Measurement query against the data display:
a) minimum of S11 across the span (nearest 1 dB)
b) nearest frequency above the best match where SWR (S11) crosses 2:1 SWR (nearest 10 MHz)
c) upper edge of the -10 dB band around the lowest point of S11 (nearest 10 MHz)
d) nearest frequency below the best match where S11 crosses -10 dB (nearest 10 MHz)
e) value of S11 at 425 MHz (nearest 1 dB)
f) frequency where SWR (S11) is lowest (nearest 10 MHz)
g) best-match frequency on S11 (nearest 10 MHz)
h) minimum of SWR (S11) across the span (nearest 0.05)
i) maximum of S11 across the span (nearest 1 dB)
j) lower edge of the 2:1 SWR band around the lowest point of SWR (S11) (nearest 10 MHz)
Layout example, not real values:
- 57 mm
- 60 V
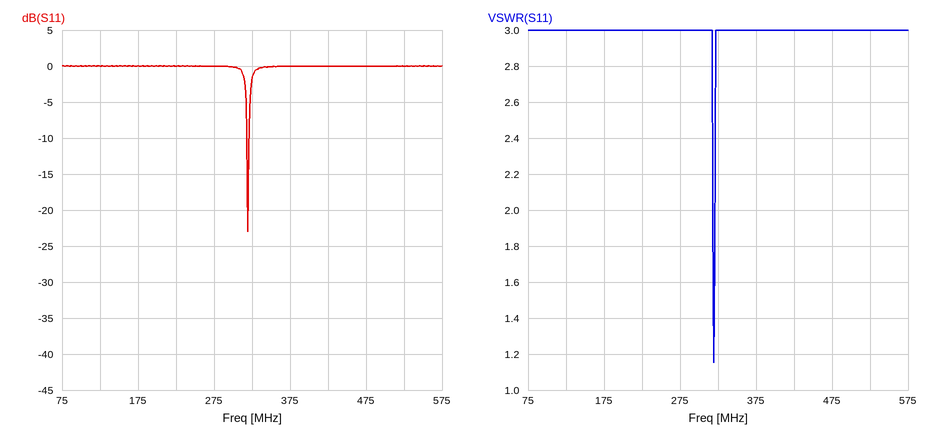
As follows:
- -23 dB
- 320 MHz
- 320 MHz
- 320 MHz
- 0 dB
- 320 MHz
- 320 MHz
- 1.15
- 0 dB
- 320 MHz
